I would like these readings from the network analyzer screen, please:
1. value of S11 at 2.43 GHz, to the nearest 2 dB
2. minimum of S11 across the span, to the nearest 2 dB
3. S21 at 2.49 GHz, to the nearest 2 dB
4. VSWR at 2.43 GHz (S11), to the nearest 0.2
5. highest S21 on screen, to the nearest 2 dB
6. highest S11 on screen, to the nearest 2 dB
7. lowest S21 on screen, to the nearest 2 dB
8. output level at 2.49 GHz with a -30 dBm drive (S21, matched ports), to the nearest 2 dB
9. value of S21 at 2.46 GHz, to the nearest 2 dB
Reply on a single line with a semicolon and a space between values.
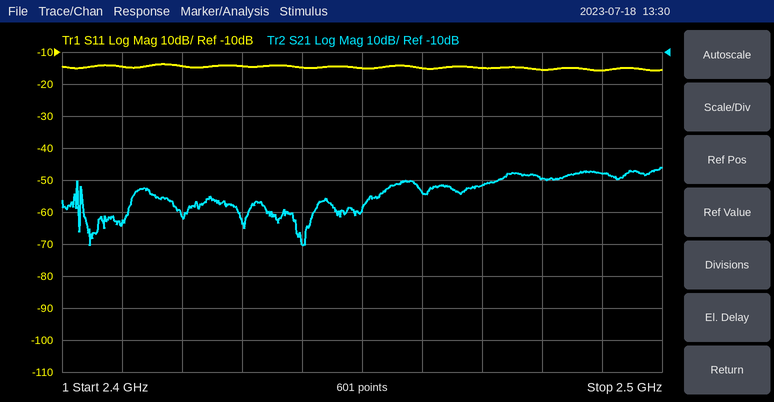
-14 dB; -16 dB; -48 dB; 1.4; -46 dB; -14 dB; -70 dB; -78 dBm; -54 dB
